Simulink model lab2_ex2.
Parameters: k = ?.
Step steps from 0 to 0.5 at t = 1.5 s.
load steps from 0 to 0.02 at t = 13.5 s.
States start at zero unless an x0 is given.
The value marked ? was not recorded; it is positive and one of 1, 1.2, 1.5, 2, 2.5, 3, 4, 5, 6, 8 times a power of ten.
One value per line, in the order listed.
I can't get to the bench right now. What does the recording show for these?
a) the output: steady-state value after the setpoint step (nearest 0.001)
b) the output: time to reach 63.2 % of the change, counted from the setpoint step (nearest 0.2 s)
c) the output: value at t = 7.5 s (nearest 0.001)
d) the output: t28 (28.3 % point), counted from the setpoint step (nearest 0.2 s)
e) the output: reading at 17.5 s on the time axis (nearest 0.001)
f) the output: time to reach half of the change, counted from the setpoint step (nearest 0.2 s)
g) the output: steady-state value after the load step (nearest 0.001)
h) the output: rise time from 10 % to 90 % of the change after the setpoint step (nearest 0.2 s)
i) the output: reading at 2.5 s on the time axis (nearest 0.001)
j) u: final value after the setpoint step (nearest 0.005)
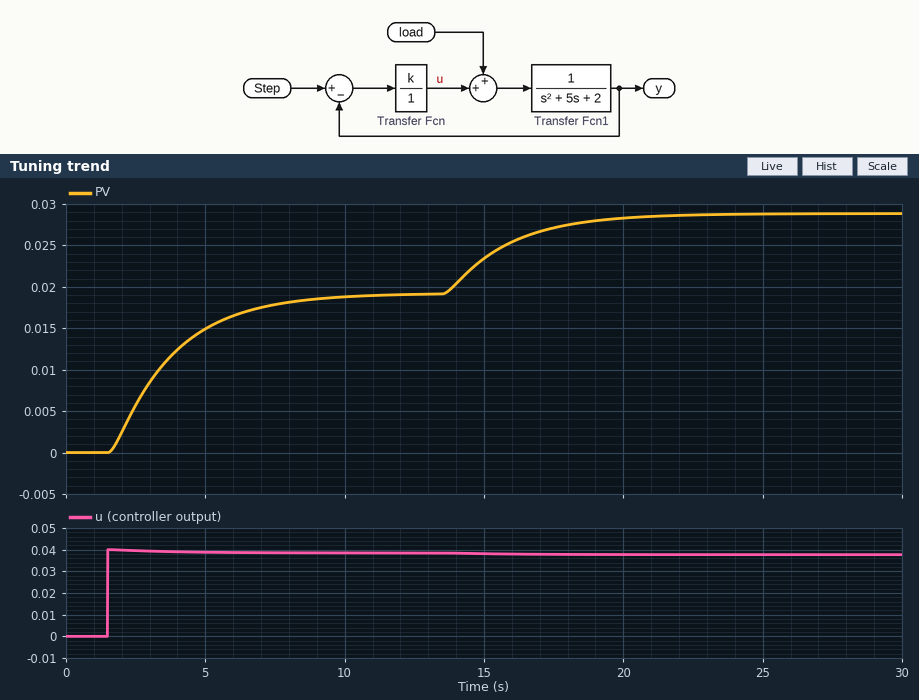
0.019
2.4 s
0.018
1.0 s
0.027
1.8 s
0.029
4.8 s
0.006
0.040
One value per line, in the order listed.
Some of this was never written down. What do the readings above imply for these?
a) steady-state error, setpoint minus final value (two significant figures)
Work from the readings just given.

0.48
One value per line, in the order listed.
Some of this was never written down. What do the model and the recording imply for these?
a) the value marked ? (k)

0.08
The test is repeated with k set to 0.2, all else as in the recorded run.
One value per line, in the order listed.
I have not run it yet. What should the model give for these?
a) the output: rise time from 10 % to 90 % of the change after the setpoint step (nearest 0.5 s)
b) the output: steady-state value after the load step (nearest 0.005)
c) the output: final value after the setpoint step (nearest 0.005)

4.5 s
0.055
0.045
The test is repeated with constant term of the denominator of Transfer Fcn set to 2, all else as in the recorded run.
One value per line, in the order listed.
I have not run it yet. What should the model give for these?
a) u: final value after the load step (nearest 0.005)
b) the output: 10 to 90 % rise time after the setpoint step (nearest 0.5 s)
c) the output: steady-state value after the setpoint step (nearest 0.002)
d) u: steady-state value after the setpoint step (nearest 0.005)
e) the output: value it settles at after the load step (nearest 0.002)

0.020
5.0 s
0.010
0.020
0.020
